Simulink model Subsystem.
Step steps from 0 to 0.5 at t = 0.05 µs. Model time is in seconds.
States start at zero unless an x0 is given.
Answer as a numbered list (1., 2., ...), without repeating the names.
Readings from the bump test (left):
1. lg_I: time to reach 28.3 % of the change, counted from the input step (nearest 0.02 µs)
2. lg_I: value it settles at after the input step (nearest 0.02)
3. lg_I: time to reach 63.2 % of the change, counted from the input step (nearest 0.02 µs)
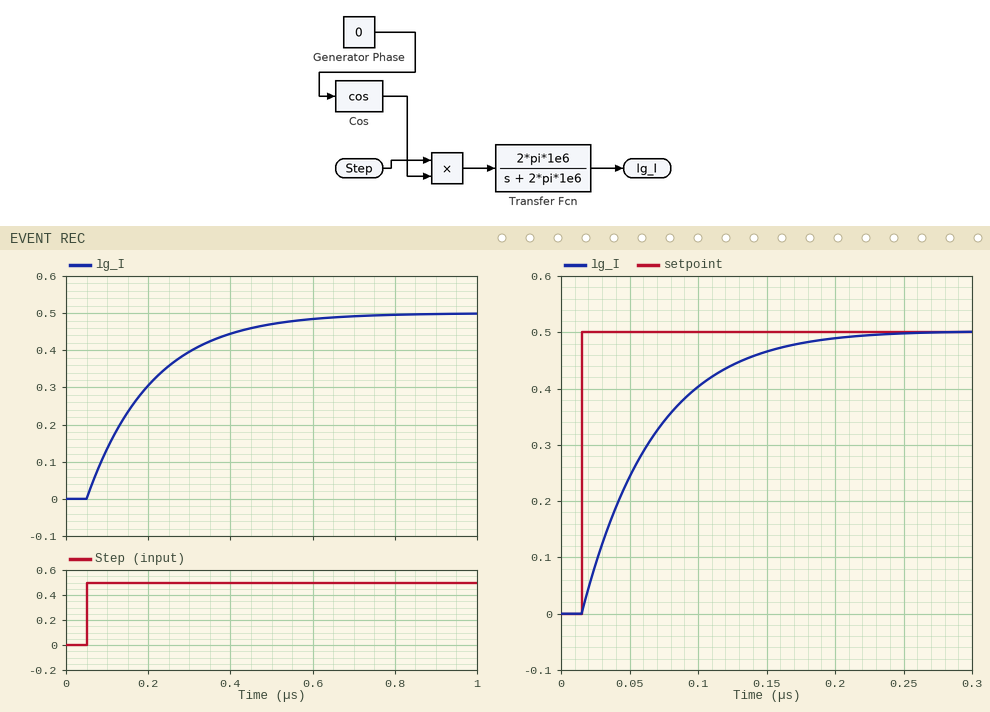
1. 0.06 µs
2. 0.50
3. 0.16 µs
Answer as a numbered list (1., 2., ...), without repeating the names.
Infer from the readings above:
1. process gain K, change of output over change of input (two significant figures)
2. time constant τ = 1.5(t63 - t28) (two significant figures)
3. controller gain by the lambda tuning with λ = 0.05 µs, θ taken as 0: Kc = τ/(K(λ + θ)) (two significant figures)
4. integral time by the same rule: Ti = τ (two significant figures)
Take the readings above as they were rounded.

1. 1.0
2. 0.15 µs
3. 3.0
4. 0.15 µs
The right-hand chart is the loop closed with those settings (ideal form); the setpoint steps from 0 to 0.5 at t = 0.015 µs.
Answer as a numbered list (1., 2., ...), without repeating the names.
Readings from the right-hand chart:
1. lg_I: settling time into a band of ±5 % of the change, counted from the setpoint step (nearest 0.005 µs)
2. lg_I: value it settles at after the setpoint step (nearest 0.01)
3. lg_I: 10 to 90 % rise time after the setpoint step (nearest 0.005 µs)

1. 0.150 µs
2. 0.50
3. 0.110 µs
